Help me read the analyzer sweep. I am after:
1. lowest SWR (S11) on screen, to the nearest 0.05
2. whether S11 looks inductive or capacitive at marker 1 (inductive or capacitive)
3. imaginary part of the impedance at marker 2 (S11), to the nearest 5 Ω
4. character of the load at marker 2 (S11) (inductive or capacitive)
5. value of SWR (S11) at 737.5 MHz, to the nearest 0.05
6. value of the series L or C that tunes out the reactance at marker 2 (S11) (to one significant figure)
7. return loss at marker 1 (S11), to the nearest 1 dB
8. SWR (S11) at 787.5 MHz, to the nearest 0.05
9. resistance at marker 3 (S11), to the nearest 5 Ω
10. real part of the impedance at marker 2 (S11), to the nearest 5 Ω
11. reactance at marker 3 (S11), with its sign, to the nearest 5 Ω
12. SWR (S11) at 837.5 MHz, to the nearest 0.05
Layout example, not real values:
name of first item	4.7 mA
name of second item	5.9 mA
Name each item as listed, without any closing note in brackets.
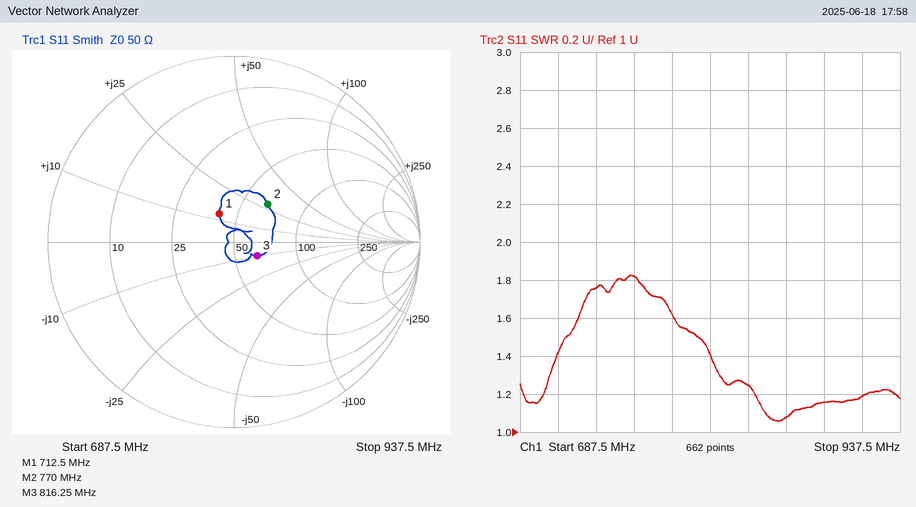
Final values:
lowest SWR (S11) on screen, to the nearest 0.05	1.05
whether S11 looks inductive or capacitive at marker 1	inductive
imaginary part of the impedance at marker 2 (S11), to the nearest 5 Ω	+30 Ω
character of the load at marker 2 (S11)	inductive
value of SWR (S11) at 737.5 MHz, to the nearest 0.05	1.75
value of the series L or C that tunes out the reactance at marker 2 (S11)	7 pF
return loss at marker 1 (S11), to the nearest 1 dB	15 dB
SWR (S11) at 787.5 MHz, to the nearest 0.05	1.60
resistance at marker 3 (S11), to the nearest 5 Ω	65 Ω
real part of the impedance at marker 2 (S11), to the nearest 5 Ω	65 Ω
reactance at marker 3 (S11), with its sign, to the nearest 5 Ω	-10 Ω
SWR (S11) at 837.5 MHz, to the nearest 0.05	1.25
